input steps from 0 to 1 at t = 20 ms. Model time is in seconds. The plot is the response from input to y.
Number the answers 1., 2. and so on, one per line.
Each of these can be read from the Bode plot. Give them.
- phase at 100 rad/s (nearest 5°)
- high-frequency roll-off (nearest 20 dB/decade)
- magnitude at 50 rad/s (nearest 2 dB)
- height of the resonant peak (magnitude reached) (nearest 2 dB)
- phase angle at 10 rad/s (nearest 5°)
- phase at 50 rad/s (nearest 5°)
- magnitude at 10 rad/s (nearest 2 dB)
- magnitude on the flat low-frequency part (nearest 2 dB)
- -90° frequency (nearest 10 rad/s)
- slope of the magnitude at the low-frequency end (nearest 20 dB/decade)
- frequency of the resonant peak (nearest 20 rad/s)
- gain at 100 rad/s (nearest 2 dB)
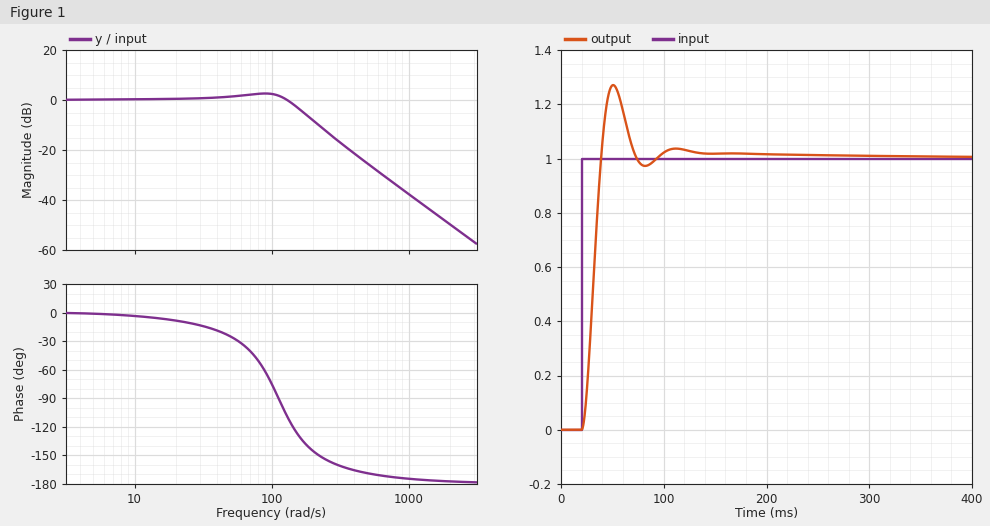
1. -75°
2. -40 dB/decade
3. 2 dB
4. 2 dB
5. -5°
6. -25°
7. 0 dB
8. 0 dB
9. 110 rad/s
10. 0 dB/decade
11. 80 rad/s
12. 2 dB
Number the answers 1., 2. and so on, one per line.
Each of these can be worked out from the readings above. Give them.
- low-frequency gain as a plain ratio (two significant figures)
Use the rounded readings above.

1. 1.0
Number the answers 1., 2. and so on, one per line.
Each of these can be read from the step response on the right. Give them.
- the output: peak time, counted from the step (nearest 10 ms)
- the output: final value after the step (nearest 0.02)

1. 30 ms
2. 1.00
